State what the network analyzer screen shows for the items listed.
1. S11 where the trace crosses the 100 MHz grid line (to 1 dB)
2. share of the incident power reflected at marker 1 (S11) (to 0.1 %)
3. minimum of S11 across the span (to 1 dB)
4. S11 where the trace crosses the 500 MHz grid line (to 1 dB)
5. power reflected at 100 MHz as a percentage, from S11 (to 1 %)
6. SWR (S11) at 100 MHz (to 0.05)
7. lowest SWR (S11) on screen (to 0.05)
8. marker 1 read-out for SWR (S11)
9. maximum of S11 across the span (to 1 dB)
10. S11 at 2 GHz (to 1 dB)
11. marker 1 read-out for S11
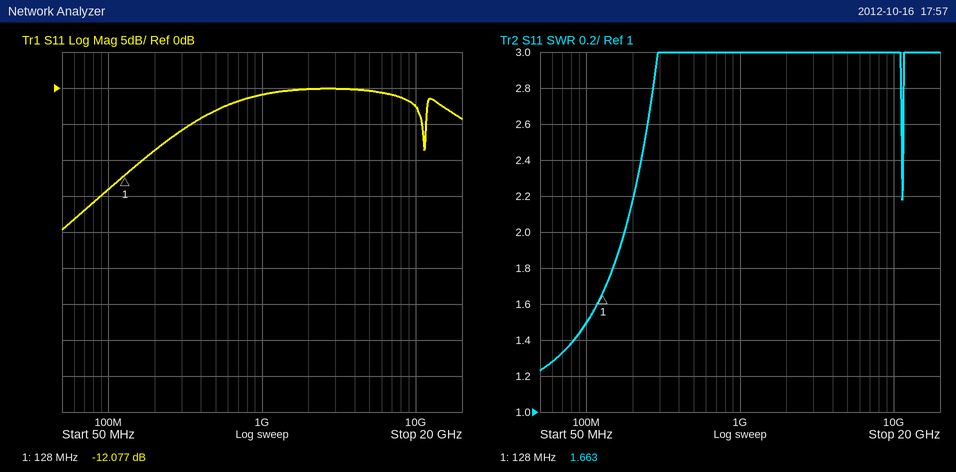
-14 dB
6.2 %
-20 dB
-3 dB
4 %
1.50
1.25
1.663
0 dB
0 dB
-12.077 dB
